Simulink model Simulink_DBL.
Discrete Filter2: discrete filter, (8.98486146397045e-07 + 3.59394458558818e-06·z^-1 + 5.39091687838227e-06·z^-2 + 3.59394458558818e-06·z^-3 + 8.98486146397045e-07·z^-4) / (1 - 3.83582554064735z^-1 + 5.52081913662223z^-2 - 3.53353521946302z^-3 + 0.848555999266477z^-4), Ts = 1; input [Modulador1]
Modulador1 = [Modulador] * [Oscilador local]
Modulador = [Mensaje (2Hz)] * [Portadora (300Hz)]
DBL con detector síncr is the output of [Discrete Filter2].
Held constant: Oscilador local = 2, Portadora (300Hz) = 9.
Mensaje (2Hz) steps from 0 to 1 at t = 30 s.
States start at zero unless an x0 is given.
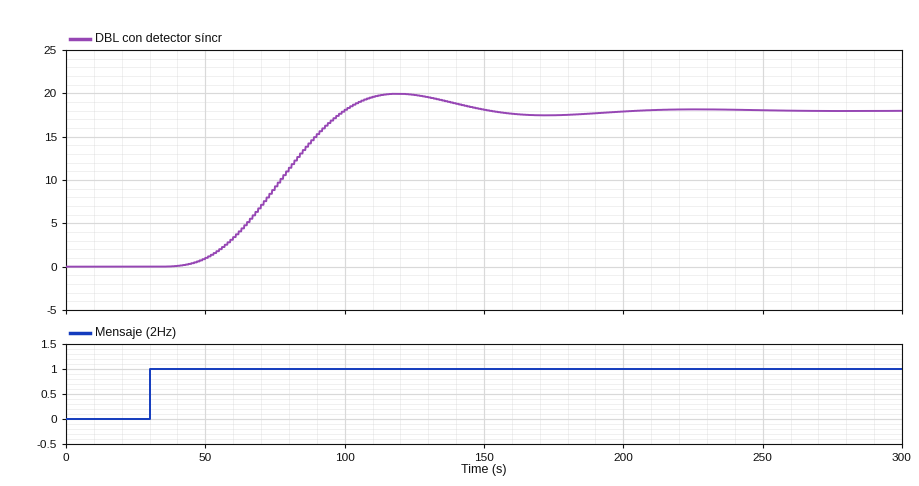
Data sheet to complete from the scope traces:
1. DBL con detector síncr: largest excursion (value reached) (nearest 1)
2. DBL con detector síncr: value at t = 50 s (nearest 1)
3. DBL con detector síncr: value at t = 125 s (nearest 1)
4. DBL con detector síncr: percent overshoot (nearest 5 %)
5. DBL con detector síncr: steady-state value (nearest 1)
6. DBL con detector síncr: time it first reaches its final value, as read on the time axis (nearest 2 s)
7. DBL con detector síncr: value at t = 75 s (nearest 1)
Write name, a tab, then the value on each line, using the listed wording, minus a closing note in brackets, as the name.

DBL con detector síncr: largest excursion (value reached)	20
DBL con detector síncr: value at t = 50 s	1
DBL con detector síncr: value at t = 125 s	20
DBL con detector síncr: percent overshoot	10 %
DBL con detector síncr: steady-state value	18
DBL con detector síncr: time it first reaches its final value, as read on the time axis	100 s
DBL con detector síncr: value at t = 75 s	9
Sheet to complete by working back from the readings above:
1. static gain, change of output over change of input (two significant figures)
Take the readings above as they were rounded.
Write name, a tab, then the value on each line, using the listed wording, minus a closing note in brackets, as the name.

static gain, change of output over change of input	18
